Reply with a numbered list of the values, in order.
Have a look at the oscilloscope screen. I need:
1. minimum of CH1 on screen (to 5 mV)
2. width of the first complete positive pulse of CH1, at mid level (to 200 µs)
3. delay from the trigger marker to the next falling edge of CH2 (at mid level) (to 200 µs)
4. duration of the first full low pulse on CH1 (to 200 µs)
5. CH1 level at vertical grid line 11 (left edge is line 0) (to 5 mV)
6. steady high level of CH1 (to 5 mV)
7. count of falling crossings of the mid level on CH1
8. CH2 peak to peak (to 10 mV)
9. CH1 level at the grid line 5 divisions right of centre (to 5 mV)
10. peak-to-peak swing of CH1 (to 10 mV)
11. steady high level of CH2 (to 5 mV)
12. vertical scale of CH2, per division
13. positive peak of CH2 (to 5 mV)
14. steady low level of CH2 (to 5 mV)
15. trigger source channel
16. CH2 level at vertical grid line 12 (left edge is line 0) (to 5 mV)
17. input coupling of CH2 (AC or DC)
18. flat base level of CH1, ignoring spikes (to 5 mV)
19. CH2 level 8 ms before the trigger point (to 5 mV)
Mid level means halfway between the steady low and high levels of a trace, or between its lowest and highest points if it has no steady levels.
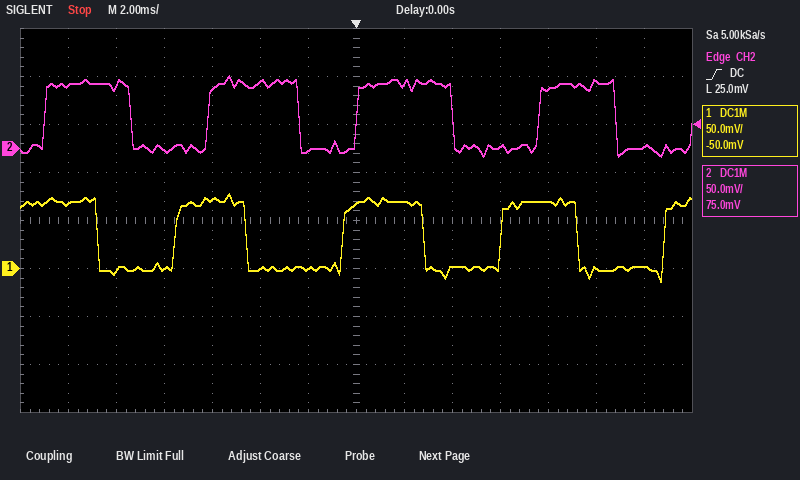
1. -15 mV
2. 3.0 ms
3. 4.0 ms
4. 3.2 ms
5. 70 mV
6. 70 mV
7. 4
8. 80 mV
9. 0 mV
10. 90 mV
11. 70 mV
12. 50 mV
13. 75 mV
14. 0 mV
15. CH2
16. 70 mV
17. DC
18. 0 mV
19. 0 mV
